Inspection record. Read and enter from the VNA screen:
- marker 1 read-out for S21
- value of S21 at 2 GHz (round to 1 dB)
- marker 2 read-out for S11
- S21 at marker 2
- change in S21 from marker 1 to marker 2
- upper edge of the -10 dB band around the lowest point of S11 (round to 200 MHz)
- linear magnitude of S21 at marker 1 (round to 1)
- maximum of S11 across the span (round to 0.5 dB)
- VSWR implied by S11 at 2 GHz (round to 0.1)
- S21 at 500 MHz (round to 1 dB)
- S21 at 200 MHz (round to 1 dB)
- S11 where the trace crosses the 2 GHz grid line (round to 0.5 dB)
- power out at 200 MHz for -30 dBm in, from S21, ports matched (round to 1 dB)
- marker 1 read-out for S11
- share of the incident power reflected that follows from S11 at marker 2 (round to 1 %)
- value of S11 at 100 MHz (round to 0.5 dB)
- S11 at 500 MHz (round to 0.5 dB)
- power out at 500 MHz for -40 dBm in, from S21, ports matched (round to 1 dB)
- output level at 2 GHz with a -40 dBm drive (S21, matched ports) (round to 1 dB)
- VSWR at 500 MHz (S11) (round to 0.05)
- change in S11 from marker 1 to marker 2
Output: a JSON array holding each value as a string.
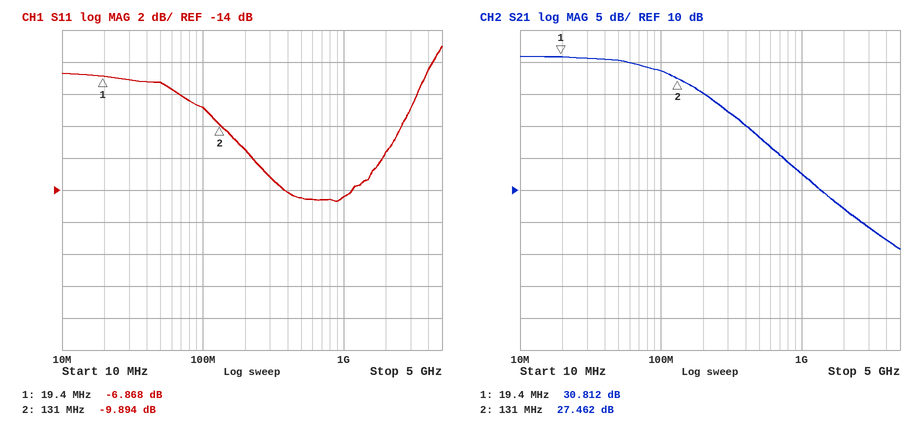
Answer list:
["30.812 dB", "7 dB", "-9.894 dB", "27.462 dB", "-3.350 dB", "2.6 GHz", "35", "-5.0 dB", "1.7", "18 dB", "25 dB", "-11.5 dB", "-5 dBm", "-6.868 dB", "10 %", "-9.0 dB", "-14.5 dB", "-22 dBm", "-33 dBm", "1.45", "-3.026 dB"]
